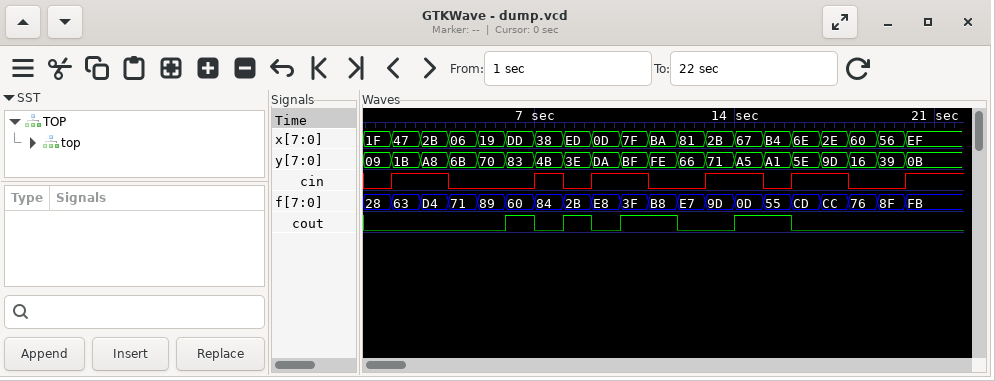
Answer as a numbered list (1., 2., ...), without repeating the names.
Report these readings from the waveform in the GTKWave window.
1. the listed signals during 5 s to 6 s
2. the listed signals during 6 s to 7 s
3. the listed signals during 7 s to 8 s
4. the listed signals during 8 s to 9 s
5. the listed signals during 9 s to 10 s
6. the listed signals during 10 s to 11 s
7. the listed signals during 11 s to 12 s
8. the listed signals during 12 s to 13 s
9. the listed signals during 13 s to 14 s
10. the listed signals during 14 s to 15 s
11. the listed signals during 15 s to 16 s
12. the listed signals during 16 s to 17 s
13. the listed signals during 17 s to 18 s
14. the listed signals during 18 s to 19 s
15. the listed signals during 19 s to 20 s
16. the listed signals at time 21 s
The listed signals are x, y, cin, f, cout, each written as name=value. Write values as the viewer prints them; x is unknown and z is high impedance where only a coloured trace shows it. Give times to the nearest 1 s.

1. x=19, y=70, cin=0, f=89, cout=0
2. x=DD, y=83, cin=0, f=60, cout=1
3. x=38, y=4B, cin=1, f=84, cout=0
4. x=ED, y=3E, cin=0, f=2B, cout=1
5. x=0D, y=DA, cin=1, f=E8, cout=0
6. x=7F, y=BF, cin=1, f=3F, cout=1
7. x=BA, y=FE, cin=0, f=B8, cout=1
8. x=81, y=66, cin=0, f=E7, cout=0
9. x=2B, y=71, cin=1, f=9D, cout=0
10. x=67, y=A5, cin=1, f=0D, cout=1
11. x=B4, y=A1, cin=0, f=55, cout=1
12. x=6E, y=5E, cin=1, f=CD, cout=0
13. x=2E, y=9D, cin=1, f=CC, cout=0
14. x=60, y=16, cin=0, f=76, cout=0
15. x=56, y=39, cin=0, f=8F, cout=0
16. x=EF, y=0B, cin=1, f=FB, cout=0
